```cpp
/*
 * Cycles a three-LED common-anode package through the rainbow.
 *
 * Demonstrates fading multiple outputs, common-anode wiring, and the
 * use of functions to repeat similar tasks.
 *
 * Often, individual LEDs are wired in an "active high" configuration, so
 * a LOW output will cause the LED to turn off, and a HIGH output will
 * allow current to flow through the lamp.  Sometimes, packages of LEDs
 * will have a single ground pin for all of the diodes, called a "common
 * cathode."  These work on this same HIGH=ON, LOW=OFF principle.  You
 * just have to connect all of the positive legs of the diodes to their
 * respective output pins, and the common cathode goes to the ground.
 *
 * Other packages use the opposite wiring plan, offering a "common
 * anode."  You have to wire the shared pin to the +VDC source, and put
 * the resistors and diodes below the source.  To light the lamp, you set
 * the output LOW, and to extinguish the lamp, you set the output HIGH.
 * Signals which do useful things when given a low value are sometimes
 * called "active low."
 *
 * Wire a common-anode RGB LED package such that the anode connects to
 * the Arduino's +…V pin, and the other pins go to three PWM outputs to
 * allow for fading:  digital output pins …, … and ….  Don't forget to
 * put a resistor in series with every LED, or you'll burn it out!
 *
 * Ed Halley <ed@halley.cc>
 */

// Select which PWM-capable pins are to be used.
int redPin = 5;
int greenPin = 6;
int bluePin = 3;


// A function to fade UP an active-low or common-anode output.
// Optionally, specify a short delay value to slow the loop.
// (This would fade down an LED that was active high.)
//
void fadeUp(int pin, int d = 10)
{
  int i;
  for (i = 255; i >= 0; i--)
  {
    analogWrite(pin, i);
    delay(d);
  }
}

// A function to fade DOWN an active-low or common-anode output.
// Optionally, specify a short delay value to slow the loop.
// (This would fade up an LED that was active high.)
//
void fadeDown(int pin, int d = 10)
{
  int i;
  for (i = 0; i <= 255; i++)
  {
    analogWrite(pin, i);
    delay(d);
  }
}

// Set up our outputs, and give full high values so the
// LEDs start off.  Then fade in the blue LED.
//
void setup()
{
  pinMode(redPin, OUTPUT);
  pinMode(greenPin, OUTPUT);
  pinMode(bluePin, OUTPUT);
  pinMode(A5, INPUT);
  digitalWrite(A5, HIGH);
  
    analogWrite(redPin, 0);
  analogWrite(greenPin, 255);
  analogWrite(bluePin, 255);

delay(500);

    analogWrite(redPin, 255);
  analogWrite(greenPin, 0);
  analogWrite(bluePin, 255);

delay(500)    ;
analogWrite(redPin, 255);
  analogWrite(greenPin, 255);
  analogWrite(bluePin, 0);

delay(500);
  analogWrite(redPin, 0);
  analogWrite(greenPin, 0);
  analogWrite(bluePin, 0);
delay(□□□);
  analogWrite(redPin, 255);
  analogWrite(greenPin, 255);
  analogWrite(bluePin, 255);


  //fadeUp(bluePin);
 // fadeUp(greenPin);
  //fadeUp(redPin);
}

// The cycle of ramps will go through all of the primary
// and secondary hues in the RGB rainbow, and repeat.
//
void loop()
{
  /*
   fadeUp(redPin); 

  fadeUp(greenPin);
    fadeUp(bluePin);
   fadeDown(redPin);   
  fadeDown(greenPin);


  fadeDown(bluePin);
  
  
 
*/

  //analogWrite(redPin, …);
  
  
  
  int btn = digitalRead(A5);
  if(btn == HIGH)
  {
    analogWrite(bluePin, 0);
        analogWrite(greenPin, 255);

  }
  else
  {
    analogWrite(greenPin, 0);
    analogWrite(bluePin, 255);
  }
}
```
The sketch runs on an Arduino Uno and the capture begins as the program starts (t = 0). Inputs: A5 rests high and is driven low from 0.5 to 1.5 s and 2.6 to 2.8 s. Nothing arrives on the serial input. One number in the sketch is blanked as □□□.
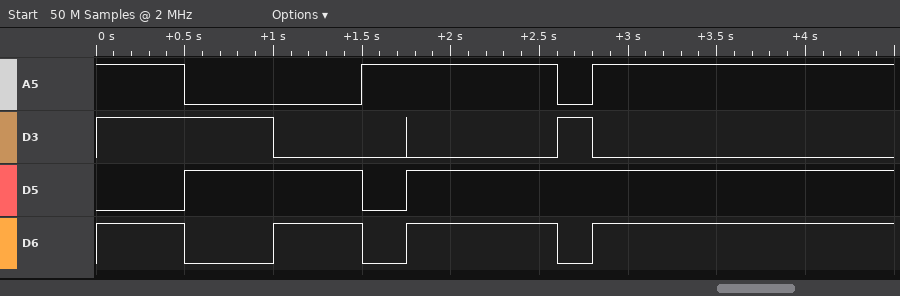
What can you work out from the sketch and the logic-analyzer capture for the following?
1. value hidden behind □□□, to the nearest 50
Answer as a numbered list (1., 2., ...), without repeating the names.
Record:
1. 250
